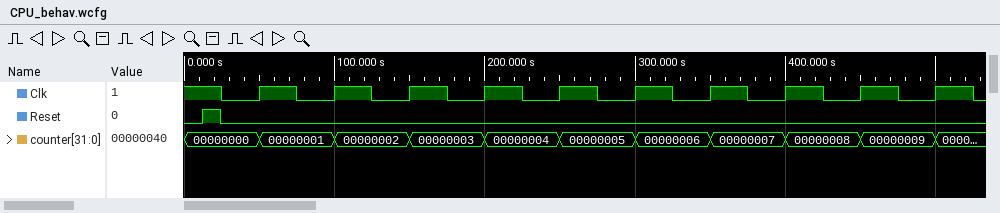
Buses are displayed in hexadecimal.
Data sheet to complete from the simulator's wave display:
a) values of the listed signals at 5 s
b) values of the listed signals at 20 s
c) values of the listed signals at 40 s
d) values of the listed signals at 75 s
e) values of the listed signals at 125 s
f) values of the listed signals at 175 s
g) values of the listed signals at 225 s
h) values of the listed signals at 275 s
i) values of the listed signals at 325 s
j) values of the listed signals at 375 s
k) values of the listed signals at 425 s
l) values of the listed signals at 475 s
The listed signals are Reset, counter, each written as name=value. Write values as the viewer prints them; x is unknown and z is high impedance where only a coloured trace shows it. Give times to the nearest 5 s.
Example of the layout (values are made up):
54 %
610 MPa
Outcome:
Reset=0, counter=00000000
Reset=1, counter=00000000
Reset=0, counter=00000000
Reset=0, counter=00000001
Reset=0, counter=00000002
Reset=0, counter=00000003
Reset=0, counter=00000004
Reset=0, counter=00000005
Reset=0, counter=00000006
Reset=0, counter=00000007
Reset=0, counter=00000008
Reset=0, counter=00000009
